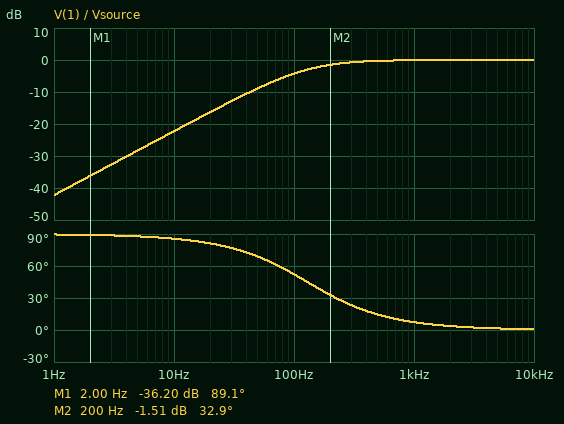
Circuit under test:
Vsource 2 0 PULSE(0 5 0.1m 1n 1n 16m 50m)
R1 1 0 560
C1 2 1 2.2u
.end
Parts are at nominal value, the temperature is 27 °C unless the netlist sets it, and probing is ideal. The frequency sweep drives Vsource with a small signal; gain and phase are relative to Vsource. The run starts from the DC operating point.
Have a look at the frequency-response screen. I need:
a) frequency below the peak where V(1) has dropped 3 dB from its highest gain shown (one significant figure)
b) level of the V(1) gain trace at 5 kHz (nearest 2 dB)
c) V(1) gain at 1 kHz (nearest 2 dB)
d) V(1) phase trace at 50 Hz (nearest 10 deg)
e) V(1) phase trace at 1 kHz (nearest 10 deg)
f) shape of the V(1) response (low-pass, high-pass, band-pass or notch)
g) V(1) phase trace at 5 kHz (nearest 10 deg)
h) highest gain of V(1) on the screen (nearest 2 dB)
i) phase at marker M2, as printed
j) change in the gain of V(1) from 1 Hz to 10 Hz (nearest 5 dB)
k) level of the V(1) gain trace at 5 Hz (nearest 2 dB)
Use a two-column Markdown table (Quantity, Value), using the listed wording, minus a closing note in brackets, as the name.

| Quantity | Value |
|---|---|
| frequency below the peak where V(1) has dropped 3 dB from its highest gain shown | 100 Hz |
| level of the V(1) gain trace at 5 kHz | 0 dB |
| V(1) gain at 1 kHz | 0 dB |
| V(1) phase trace at 50 Hz | 70 deg |
| V(1) phase trace at 1 kHz | 10 deg |
| shape of the V(1) response | high-pass |
| V(1) phase trace at 5 kHz | 0 deg |
| highest gain of V(1) on the screen | 0 dB |
| phase at marker M2, as printed | 32.9 deg |
| change in the gain of V(1) from 1 Hz to 10 Hz | 20 dB |
| level of the V(1) gain trace at 5 Hz | -28 dB |
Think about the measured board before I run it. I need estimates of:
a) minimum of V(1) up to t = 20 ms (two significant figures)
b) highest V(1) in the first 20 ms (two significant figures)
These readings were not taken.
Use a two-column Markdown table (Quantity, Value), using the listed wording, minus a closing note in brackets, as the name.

| Quantity | Value |
|---|---|
| minimum of V(1) up to t = 20 ms | -5.0 V |
| highest V(1) in the first 20 ms | 5.0 V |
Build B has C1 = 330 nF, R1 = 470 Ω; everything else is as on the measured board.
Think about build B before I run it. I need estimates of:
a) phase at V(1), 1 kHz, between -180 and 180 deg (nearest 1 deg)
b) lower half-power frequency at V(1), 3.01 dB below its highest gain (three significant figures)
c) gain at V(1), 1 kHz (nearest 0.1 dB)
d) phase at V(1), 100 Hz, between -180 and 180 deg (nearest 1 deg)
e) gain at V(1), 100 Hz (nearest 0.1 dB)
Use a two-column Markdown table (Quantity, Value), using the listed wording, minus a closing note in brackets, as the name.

| Quantity | Value |
|---|---|
| phase at V(1), 1 kHz, between -180 and 180 deg | 46 deg |
| lower half-power frequency at V(1), 3.01 dB below its highest gain | 1.03 kHz |
| gain at V(1), 1 kHz | -3.1 dB |
| phase at V(1), 100 Hz, between -180 and 180 deg | 84 deg |
| gain at V(1), 100 Hz | -20.3 dB |
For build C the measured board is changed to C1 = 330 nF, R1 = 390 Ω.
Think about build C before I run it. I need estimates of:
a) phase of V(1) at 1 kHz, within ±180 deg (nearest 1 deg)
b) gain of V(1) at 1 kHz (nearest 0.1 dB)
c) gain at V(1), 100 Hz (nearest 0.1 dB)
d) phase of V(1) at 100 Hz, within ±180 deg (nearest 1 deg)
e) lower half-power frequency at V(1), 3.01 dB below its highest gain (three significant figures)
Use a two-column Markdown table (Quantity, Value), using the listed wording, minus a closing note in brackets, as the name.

| Quantity | Value |
|---|---|
| phase of V(1) at 1 kHz, within ±180 deg | 51 deg |
| gain of V(1) at 1 kHz | -4.0 dB |
| gain at V(1), 100 Hz | -21.9 dB |
| phase of V(1) at 100 Hz, within ±180 deg | 85 deg |
| lower half-power frequency at V(1), 3.01 dB below its highest gain | 1.24 kHz |
